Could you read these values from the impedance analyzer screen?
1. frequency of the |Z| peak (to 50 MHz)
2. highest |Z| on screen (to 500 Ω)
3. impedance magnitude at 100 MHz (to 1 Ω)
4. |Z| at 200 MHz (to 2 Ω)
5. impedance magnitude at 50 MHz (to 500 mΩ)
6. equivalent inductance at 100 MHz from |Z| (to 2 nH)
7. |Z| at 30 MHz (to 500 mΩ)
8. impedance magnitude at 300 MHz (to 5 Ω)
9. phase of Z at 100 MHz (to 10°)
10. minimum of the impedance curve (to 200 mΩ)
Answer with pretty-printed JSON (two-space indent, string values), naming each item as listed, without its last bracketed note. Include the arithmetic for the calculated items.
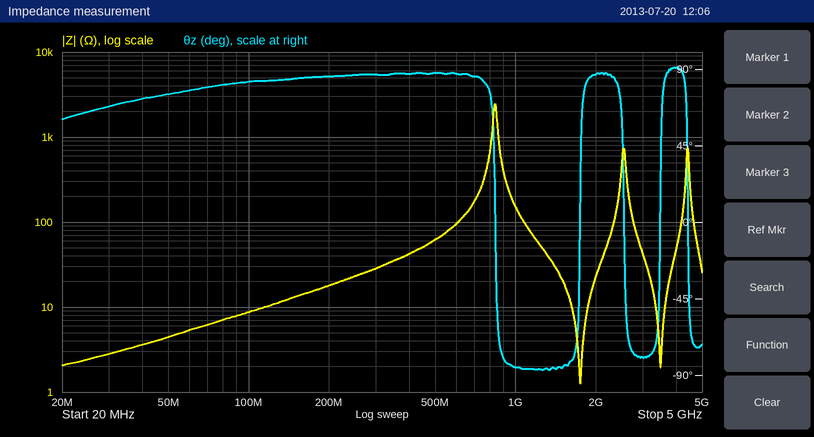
{
  "frequency of the |Z| peak": "850 MHz",
  "highest |Z| on screen": "2.5 kΩ",
  "impedance magnitude at 100 MHz": "9 Ω",
  "|Z| at 200 MHz": "18 Ω",
  "impedance magnitude at 50 MHz": "4.5 Ω",
  "equivalent inductance at 100 MHz from |Z|": "L = 9 Ω/(2π × 100 MHz) ≈ 14 nH",
  "|Z| at 30 MHz": "3.0 Ω",
  "impedance magnitude at 300 MHz": "30 Ω",
  "phase of Z at 100 MHz": "80°",
  "minimum of the impedance curve": "1.2 Ω"
}
